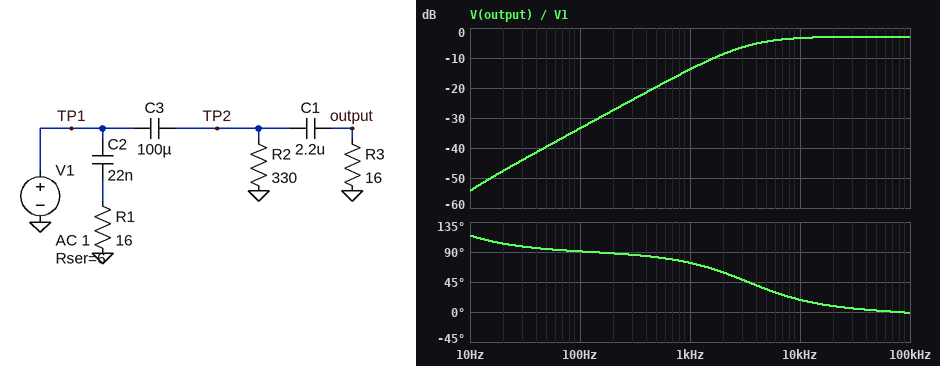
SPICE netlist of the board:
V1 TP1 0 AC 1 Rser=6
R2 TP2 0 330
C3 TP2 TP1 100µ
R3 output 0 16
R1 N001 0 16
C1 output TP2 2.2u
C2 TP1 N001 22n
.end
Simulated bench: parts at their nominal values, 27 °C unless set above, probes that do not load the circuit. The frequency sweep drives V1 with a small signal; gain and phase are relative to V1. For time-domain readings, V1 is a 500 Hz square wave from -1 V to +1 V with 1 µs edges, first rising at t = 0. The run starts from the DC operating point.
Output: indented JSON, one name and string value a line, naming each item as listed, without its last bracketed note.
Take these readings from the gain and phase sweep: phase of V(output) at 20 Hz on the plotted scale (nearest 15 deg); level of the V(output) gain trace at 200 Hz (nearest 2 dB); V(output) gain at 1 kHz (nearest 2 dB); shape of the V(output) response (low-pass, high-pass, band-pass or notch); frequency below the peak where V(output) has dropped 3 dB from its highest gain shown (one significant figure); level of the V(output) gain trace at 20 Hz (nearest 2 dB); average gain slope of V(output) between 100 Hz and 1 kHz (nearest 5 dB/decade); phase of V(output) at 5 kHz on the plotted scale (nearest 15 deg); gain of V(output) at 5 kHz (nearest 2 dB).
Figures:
{
  "phase of V(output) at 20 Hz on the plotted scale": "105 deg",
  "level of the V(output) gain trace at 200 Hz": "-28 dB",
  "V(output) gain at 1 kHz": "-14 dB",
  "shape of the V(output) response": "high-pass",
  "frequency below the peak where V(output) has dropped 3 dB from its highest gain shown": "3 kHz",
  "level of the V(output) gain trace at 20 Hz": "-48 dB",
  "average gain slope of V(output) between 100 Hz and 1 kHz": "20 dB/decade",
  "phase of V(output) at 5 kHz on the plotted scale": "30 deg",
  "gain of V(output) at 5 kHz": "-4 dB"
}
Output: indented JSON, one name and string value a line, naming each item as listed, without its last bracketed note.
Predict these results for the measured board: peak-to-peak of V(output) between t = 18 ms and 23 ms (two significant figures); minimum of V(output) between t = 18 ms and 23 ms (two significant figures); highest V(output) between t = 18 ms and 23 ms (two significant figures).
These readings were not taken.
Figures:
{
  "peak-to-peak of V(output) between t = 18 ms and 23 ms": "2.8 V",
  "minimum of V(output) between t = 18 ms and 23 ms": "-1.4 V",
  "highest V(output) between t = 18 ms and 23 ms": "1.4 V"
}
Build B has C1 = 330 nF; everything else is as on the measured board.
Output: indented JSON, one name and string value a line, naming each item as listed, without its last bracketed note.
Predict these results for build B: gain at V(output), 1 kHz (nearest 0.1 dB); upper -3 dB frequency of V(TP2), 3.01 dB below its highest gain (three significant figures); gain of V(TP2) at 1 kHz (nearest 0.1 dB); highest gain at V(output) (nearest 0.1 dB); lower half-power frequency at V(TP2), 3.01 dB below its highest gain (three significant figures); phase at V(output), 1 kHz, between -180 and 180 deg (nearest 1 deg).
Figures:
{
  "gain at V(output), 1 kHz": "-29.8 dB",
  "upper -3 dB frequency of V(TP2), 3.01 dB below its highest gain": "177 kHz",
  "gain of V(TP2) at 1 kHz": "-0.2 dB",
  "highest gain at V(output)": "-3.2 dB",
  "lower half-power frequency at V(TP2), 3.01 dB below its highest gain": "4.72 Hz",
  "phase at V(output), 1 kHz, between -180 and 180 deg": "88 deg"
}
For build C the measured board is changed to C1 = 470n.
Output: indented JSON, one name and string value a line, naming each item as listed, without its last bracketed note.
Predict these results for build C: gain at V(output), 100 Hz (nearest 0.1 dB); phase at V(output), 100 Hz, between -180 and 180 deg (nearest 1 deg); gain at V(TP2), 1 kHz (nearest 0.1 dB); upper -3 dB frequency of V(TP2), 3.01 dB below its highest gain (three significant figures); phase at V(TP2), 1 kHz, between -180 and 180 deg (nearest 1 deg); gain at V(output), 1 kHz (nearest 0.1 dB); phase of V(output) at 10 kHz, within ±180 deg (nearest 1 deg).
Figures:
{
  "gain at V(output), 100 Hz": "-46.7 dB",
  "phase at V(output), 100 Hz, between -180 and 180 deg": "92 deg",
  "gain at V(TP2), 1 kHz": "-0.2 dB",
  "upper -3 dB frequency of V(TP2), 3.01 dB below its highest gain": "175 kHz",
  "phase at V(TP2), 1 kHz, between -180 and 180 deg": "-1 deg",
  "gain at V(output), 1 kHz": "-26.7 dB",
  "phase of V(output) at 10 kHz, within ±180 deg": "57 deg"
}
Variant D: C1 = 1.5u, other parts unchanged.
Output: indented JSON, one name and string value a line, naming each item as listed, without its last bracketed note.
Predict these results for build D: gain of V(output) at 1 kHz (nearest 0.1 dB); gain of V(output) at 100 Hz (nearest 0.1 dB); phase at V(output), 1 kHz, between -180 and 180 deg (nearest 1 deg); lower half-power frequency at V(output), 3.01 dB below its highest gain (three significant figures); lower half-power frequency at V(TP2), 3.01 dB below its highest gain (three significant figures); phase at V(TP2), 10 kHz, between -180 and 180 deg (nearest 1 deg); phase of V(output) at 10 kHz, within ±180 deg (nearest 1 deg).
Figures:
{
  "gain of V(output) at 1 kHz": "-16.9 dB",
  "gain of V(output) at 100 Hz": "-36.7 dB",
  "phase at V(output), 1 kHz, between -180 and 180 deg": "79 deg",
  "lower half-power frequency at V(output), 3.01 dB below its highest gain": "4.83 kHz",
  "lower half-power frequency at V(TP2), 3.01 dB below its highest gain": "4.66 Hz",
  "phase at V(TP2), 10 kHz, between -180 and 180 deg": "-8 deg",
  "phase of V(output) at 10 kHz, within ±180 deg": "26 deg"
}
